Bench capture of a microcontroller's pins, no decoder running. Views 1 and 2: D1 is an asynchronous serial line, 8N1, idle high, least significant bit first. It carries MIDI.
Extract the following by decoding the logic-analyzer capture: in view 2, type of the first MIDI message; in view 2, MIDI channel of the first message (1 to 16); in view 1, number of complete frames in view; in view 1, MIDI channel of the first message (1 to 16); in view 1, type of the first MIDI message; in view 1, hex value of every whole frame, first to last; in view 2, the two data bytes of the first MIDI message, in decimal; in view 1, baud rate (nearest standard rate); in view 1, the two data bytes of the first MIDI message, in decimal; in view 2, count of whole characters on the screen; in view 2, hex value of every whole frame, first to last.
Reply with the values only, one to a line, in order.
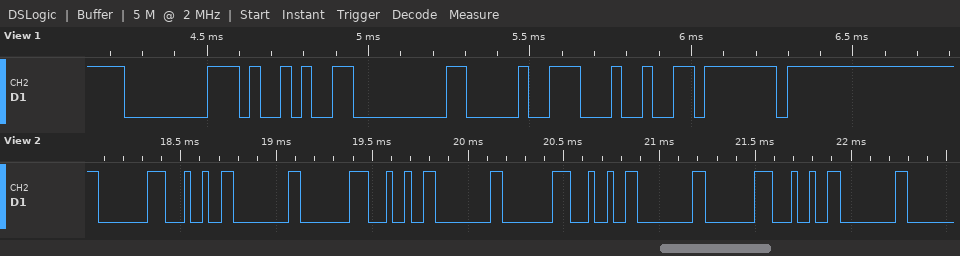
Note Off
1
6
1
Note Off
80 29 00 90 24 7F
36, 0
31250 baud
41, 0
12
80 24 00 80 24 00 80 24 00 80 24 00
